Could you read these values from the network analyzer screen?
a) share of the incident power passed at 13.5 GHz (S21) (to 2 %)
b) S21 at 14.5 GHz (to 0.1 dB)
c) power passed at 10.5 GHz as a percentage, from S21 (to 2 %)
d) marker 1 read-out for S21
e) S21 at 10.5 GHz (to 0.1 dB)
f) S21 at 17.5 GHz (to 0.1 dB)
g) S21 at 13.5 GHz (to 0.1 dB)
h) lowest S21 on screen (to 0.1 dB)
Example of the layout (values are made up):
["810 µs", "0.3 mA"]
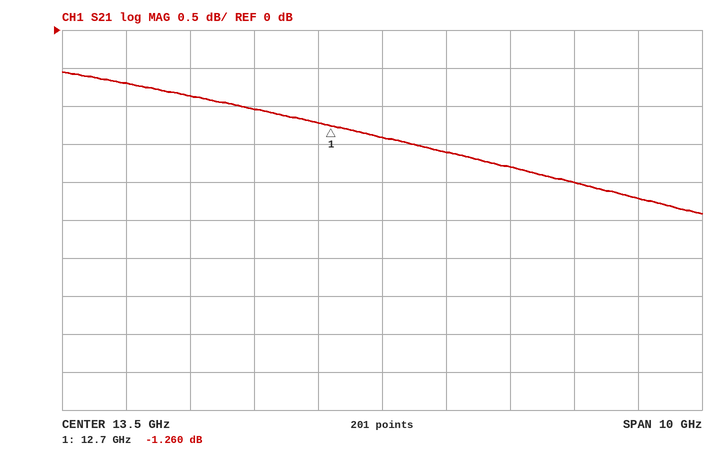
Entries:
["72 %", "-1.6 dB", "82 %", "-1.260 dB", "-0.9 dB", "-2.2 dB", "-1.4 dB", "-2.4 dB"]
